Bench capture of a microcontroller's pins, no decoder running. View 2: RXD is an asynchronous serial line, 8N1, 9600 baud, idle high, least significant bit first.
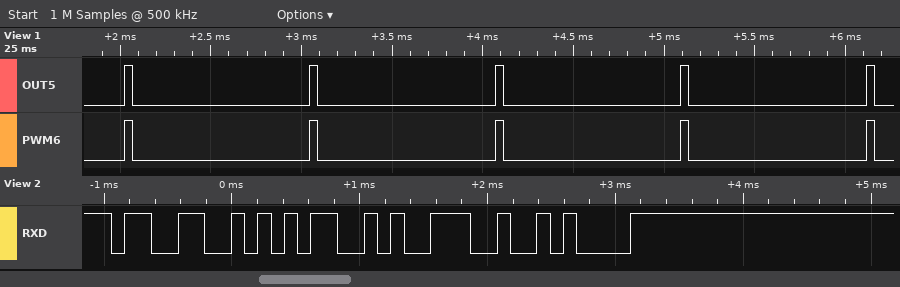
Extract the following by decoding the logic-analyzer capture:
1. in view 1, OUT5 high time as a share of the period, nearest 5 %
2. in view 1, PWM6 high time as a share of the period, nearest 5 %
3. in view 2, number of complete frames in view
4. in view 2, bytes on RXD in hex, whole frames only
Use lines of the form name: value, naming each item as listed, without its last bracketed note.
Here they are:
in view 1, OUT5 high time as a share of the period, nearest 5 %: 5 %
in view 1, PWM6 high time as a share of the period, nearest 5 %: 5 %
in view 2, number of complete frames in view: 4
in view 2, bytes on RXD in hex, whole frames only: 0x33 0x35 0x39 0x0A
